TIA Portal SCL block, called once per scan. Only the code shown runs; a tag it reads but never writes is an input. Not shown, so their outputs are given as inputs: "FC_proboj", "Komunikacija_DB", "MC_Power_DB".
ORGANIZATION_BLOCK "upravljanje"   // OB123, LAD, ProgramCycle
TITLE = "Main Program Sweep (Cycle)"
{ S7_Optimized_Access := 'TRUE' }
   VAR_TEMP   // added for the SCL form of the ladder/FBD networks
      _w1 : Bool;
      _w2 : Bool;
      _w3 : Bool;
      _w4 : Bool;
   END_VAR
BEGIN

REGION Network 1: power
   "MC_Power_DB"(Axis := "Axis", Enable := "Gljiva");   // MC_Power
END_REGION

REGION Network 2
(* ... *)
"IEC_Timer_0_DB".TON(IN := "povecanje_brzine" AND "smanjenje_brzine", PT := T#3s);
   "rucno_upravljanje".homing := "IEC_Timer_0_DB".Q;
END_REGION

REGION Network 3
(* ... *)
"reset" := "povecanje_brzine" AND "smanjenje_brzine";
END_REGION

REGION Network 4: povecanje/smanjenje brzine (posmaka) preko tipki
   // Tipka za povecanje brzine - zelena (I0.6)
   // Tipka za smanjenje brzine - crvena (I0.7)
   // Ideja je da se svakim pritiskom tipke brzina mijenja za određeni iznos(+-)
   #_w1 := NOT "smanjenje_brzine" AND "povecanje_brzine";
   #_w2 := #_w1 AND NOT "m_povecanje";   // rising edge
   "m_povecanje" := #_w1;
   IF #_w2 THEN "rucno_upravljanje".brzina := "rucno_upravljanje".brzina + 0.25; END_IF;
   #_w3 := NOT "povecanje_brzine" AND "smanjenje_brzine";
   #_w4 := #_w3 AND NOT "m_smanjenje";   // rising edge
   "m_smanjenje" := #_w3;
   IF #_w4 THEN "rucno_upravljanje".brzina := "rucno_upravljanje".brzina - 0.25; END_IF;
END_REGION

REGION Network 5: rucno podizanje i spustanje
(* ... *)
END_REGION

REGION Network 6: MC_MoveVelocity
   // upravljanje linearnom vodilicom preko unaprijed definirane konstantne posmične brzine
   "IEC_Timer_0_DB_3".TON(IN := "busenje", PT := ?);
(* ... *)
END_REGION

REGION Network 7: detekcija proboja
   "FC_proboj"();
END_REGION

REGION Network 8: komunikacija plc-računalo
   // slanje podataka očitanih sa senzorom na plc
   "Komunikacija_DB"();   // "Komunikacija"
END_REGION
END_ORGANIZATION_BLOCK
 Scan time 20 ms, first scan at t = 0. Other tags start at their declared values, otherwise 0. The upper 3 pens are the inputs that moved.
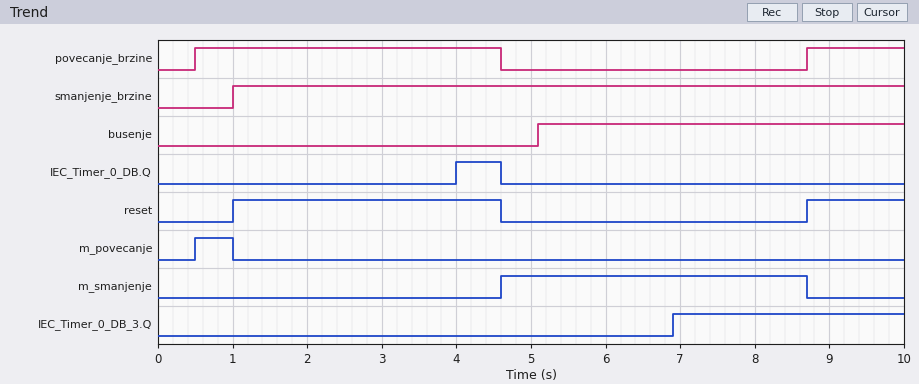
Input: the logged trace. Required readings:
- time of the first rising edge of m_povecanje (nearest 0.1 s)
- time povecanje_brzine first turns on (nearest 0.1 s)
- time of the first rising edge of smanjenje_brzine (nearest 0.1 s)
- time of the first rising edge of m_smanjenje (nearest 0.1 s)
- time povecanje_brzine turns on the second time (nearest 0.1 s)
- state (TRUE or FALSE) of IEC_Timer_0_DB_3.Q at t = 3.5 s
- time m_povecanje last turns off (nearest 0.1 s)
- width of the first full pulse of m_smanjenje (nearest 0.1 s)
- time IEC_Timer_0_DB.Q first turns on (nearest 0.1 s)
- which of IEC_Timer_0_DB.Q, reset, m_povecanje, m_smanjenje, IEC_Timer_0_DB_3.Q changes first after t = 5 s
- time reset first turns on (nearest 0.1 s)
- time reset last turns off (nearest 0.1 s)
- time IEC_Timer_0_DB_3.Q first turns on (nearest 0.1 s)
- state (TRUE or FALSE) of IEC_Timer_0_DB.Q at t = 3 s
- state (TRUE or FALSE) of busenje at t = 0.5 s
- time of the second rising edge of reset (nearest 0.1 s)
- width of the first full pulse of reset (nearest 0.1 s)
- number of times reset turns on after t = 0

0.5 s
0.5 s
1.0 s
4.6 s
8.7 s
FALSE
1.0 s
4.1 s
4.0 s
IEC_Timer_0_DB_3.Q
1.0 s
4.6 s
6.9 s
FALSE
FALSE
8.7 s
3.6 s
2
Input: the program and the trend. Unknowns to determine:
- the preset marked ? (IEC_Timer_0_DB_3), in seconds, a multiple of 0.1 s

1.8 s
